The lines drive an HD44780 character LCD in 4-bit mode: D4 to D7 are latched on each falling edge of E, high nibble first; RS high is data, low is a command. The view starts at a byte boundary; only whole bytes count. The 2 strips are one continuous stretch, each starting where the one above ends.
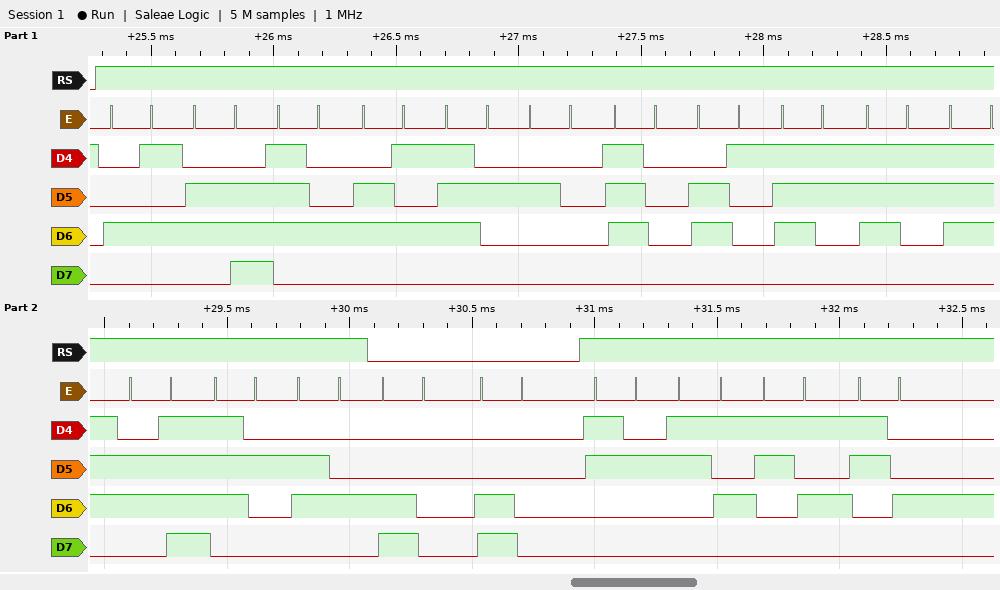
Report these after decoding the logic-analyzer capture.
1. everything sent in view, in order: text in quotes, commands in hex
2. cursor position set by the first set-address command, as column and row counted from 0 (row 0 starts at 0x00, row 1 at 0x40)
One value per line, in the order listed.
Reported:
"Enter password" 0xC0 0xC0 "2554"
column 0, row 1
